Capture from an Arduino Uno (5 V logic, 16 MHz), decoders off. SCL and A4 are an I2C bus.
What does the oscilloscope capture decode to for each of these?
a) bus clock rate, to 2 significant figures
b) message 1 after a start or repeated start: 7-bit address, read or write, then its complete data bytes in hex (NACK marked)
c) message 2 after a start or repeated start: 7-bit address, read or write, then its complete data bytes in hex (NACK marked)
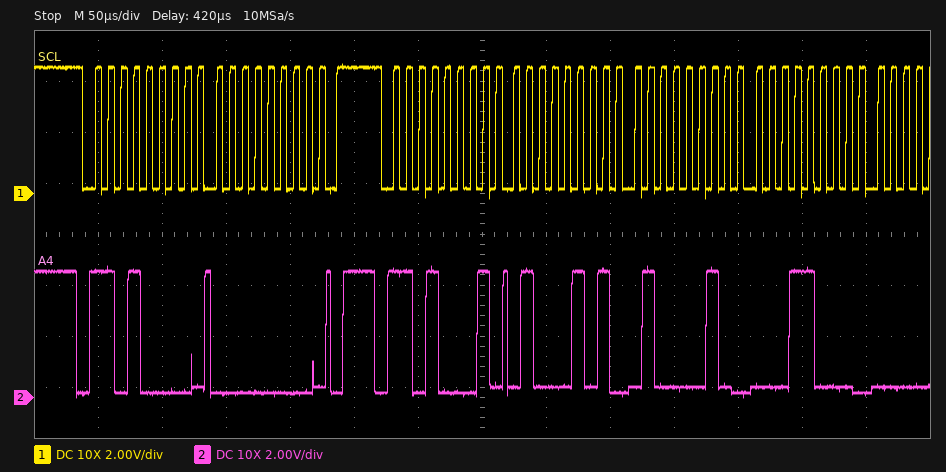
100 kHz
0x68 write: 00
0x68 read: 45 42 18
